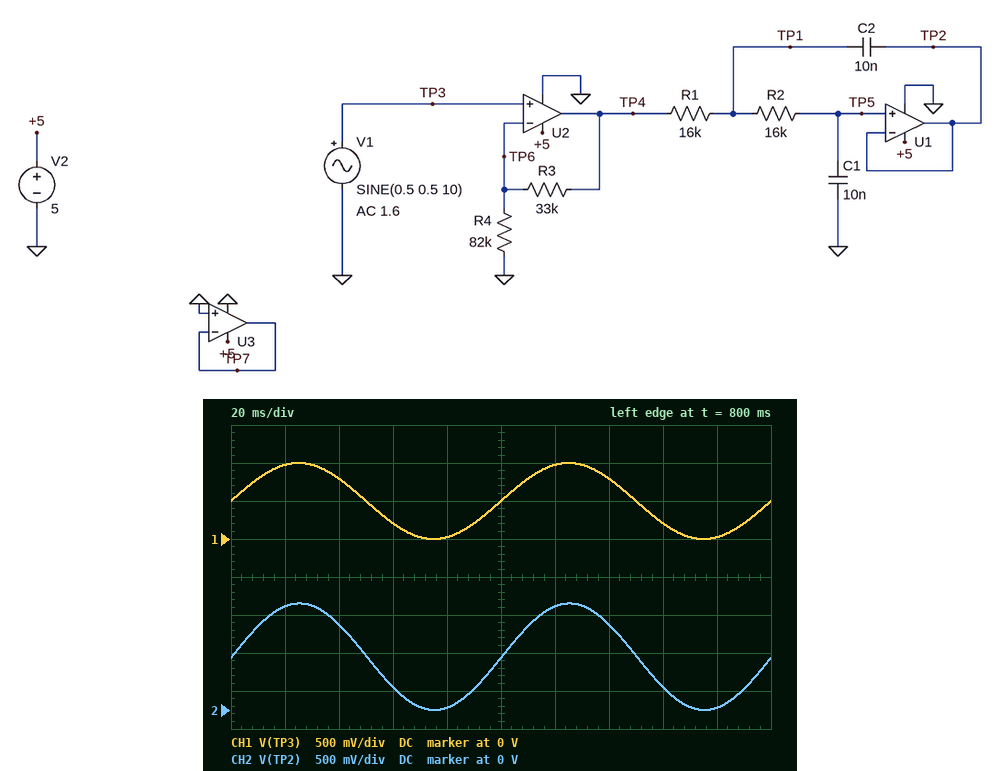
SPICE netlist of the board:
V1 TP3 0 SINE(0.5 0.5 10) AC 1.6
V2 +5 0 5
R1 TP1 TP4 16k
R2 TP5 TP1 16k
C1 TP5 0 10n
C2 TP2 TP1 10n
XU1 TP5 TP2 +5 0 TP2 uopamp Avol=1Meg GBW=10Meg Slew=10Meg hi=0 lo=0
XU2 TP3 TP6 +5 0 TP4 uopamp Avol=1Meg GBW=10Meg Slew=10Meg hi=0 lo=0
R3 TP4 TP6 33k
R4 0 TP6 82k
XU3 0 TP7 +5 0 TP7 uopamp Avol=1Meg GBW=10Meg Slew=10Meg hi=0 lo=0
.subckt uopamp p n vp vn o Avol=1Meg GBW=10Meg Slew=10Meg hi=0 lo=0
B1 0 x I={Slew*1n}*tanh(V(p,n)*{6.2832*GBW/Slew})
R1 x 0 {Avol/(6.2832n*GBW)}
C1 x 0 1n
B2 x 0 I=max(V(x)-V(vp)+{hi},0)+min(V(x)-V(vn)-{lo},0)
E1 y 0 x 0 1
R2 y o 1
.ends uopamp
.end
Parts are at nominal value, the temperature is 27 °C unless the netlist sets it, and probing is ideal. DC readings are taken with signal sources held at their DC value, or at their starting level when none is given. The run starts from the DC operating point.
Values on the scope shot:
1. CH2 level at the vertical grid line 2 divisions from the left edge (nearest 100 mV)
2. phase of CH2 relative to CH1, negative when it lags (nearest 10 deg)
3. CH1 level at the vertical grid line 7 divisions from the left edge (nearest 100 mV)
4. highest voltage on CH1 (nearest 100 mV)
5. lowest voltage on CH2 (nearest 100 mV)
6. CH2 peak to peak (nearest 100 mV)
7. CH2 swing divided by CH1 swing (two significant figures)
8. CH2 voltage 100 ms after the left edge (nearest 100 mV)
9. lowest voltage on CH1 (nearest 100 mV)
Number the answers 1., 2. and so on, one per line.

1. 1.1 V
2. 0 deg
3. 800 mV
4. 1.0 V
5. 0 V
6. 1.4 V
7. 1.4
8. 700 mV
9. 0 V
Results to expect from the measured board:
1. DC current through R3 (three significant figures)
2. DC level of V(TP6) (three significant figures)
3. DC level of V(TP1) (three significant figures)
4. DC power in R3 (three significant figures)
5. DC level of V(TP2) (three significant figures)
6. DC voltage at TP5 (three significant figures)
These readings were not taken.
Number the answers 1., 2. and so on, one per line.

1. 6.10 µA
2. 500 mV
3. 701 mV
4. 1.23 µW
5. 701 mV
6. 701 mV
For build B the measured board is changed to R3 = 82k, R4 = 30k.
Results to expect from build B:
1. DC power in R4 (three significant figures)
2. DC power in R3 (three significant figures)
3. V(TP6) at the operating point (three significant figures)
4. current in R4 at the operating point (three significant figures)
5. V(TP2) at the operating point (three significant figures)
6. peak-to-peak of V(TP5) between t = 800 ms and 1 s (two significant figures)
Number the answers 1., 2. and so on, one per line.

1. 8.33 µW
2. 22.8 µW
3. 500 mV
4. 16.7 µA
5. 1.87 V
6. 3.7 V
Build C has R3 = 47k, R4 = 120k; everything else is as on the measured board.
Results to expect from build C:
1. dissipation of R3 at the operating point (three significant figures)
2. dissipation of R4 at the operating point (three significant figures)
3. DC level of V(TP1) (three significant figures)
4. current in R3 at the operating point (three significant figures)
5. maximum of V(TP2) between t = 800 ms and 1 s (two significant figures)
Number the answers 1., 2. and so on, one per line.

1. 816 nW
2. 2.08 µW
3. 696 mV
4. 4.17 µA
5. 1.4 V
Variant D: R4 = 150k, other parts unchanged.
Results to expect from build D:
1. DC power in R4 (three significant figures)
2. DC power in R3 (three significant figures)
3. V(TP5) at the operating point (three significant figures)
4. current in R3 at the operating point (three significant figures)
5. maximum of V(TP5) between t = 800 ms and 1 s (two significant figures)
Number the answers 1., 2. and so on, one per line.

1. 1.67 µW
2. 367 nW
3. 610 mV
4. 3.33 µA
5. 1.2 V
